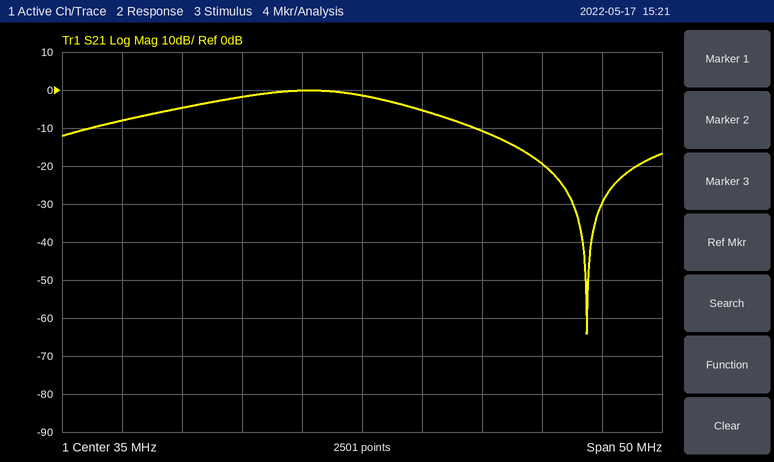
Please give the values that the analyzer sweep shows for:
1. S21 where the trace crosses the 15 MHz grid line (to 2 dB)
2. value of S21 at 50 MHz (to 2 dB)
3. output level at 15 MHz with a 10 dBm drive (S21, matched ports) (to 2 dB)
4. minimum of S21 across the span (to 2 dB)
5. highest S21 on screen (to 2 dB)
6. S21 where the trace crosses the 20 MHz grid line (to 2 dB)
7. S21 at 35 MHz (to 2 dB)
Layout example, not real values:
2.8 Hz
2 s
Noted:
-8 dB
-20 dB
2 dBm
-64 dB
0 dB
-4 dB
-2 dB
